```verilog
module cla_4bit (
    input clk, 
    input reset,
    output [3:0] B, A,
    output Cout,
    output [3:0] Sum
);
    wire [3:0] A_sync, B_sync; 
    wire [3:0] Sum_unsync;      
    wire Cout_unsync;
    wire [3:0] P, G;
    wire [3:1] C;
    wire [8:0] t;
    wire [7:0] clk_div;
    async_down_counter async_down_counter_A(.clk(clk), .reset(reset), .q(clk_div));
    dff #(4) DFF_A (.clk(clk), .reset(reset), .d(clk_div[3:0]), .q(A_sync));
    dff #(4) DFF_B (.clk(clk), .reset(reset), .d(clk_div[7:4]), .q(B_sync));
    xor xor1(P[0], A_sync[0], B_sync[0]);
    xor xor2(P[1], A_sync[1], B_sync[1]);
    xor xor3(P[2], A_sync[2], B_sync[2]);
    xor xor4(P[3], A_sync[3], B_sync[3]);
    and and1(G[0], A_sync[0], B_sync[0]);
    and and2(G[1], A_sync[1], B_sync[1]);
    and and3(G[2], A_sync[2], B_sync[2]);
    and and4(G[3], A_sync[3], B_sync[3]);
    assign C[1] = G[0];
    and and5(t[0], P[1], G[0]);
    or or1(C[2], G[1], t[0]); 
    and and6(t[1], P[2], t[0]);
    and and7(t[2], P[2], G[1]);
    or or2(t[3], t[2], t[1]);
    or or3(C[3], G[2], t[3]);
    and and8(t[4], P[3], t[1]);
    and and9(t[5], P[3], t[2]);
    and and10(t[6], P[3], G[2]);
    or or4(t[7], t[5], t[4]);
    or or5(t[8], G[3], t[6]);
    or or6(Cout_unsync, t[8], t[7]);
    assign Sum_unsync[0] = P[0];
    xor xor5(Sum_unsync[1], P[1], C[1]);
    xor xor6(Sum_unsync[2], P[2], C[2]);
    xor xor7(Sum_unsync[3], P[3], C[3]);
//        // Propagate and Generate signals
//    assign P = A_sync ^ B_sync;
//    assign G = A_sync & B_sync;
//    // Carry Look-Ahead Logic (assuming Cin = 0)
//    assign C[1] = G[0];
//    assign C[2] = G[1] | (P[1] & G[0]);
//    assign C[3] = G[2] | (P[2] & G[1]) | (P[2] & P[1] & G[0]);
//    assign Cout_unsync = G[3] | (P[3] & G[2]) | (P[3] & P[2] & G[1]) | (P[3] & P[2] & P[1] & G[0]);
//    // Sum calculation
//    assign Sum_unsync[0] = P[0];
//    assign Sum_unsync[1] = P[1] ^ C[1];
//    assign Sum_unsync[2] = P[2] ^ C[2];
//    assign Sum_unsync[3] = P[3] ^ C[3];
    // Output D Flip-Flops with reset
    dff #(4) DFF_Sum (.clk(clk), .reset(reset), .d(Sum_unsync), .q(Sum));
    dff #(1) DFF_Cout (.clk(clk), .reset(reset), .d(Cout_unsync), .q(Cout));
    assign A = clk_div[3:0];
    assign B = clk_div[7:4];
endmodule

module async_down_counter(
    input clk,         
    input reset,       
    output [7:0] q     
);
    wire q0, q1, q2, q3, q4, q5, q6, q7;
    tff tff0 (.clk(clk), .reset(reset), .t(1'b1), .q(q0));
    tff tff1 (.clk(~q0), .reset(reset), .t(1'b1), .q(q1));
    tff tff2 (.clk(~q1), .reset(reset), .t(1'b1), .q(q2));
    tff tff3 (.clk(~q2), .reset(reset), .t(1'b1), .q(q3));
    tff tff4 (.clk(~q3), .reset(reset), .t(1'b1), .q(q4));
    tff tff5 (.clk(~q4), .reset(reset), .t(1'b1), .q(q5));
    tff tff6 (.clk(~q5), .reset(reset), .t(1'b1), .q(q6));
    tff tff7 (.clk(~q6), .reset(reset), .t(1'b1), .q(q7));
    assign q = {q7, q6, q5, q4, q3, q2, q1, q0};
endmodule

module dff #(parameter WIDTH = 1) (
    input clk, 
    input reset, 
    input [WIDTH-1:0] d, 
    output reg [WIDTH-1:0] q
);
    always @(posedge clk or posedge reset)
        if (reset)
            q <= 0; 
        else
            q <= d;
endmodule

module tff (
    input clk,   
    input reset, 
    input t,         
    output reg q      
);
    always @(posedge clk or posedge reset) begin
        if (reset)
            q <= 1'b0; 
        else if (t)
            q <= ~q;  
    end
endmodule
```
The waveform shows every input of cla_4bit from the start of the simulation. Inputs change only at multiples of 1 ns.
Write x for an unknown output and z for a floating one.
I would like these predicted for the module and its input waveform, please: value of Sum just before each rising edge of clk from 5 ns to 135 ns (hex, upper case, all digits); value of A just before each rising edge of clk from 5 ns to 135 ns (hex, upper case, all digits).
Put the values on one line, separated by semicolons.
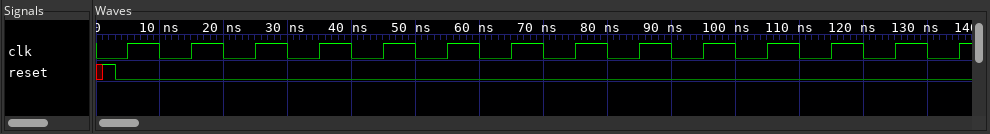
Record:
0, 0, 0, 1, 2, 3, 4, 5, 6, 7, 8, 9, A, B; 0, 1, 2, 3, 4, 5, 6, 7, 8, 9, A, B, C, D
